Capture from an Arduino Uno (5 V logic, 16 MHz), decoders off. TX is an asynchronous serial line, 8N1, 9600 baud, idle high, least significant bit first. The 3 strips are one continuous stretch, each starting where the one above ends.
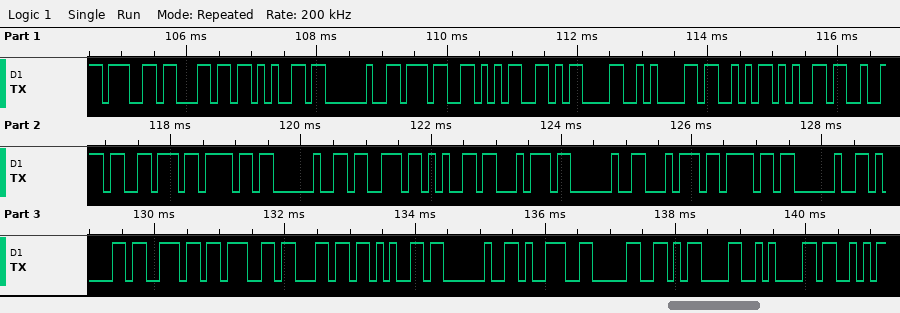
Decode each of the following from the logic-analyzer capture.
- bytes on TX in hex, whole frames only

67 6C 65 20 37 35 0D 0A 53 65 72 76 6F 20 73 65 74 20 74 6F 20 61 6E 67 6C 65 20 39 30 0D 0A 53
